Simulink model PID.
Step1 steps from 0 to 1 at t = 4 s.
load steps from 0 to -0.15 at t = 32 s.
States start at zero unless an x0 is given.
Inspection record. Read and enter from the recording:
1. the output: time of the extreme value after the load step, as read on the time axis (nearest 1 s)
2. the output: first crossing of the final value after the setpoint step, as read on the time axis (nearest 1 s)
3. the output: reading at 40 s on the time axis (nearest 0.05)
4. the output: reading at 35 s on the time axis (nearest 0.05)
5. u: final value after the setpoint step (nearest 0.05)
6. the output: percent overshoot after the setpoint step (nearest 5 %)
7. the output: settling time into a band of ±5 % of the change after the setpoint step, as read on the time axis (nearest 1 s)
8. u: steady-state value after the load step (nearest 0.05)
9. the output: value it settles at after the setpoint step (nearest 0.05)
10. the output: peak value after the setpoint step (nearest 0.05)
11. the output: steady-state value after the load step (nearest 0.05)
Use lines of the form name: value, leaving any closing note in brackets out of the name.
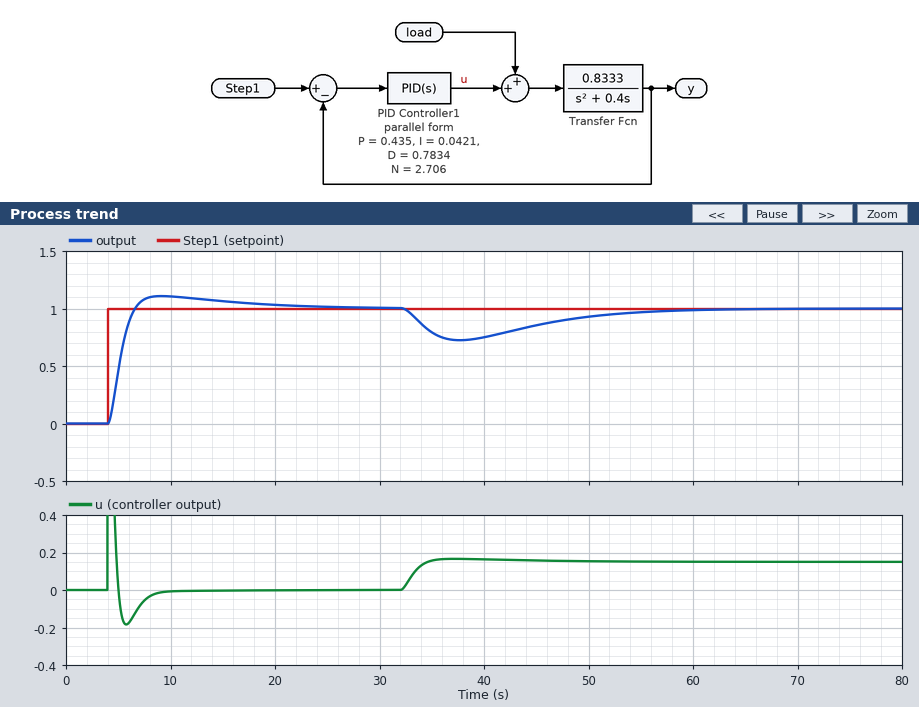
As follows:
the output: time of the extreme value after the load step, as read on the time axis: 38 s
the output: first crossing of the final value after the setpoint step, as read on the time axis: 7 s
the output: reading at 40 s on the time axis: 0.75
the output: reading at 35 s on the time axis: 0.80
u: final value after the setpoint step: 0.00
the output: percent overshoot after the setpoint step: 10 %
the output: settling time into a band of ±5 % of the change after the setpoint step, as read on the time axis: 17 s
u: steady-state value after the load step: 0.15
the output: value it settles at after the setpoint step: 1.00
the output: peak value after the setpoint step: 1.10
the output: steady-state value after the load step: 1.00
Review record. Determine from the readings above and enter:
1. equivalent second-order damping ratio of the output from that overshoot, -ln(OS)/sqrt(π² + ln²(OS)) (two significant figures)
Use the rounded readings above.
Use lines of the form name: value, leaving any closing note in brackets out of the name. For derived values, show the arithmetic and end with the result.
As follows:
equivalent second-order damping ratio of the output from that overshoot, -ln(OS)/sqrt(π² + ln²(OS)): ln(0.1) = -2.303; 2.303 / sqrt(9.870 + 5.302) = 0.59
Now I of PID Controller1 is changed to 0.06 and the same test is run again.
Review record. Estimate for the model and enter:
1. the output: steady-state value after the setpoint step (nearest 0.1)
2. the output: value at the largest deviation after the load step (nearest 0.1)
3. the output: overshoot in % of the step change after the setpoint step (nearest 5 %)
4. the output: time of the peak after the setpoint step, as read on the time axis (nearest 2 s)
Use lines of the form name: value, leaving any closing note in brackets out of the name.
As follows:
the output: steady-state value after the setpoint step: 1.0
the output: value at the largest deviation after the load step: 0.7
the output: overshoot in % of the step change after the setpoint step: 15 %
the output: time of the peak after the setpoint step, as read on the time axis: 10 s
